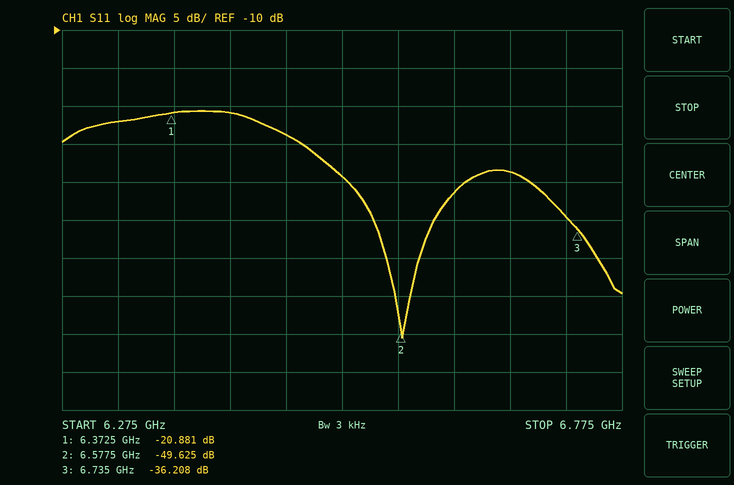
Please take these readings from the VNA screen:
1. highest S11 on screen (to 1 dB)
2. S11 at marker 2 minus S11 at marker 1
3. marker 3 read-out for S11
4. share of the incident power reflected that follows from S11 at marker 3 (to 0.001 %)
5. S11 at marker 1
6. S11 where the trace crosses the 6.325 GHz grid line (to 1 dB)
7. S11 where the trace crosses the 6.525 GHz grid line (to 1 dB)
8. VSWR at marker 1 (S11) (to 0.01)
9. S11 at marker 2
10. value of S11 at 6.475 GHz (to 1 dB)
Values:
-21 dB
-28.744 dB
-36.208 dB
0.024 %
-20.881 dB
-22 dB
-29 dB
1.20
-49.625 dB
-24 dB
